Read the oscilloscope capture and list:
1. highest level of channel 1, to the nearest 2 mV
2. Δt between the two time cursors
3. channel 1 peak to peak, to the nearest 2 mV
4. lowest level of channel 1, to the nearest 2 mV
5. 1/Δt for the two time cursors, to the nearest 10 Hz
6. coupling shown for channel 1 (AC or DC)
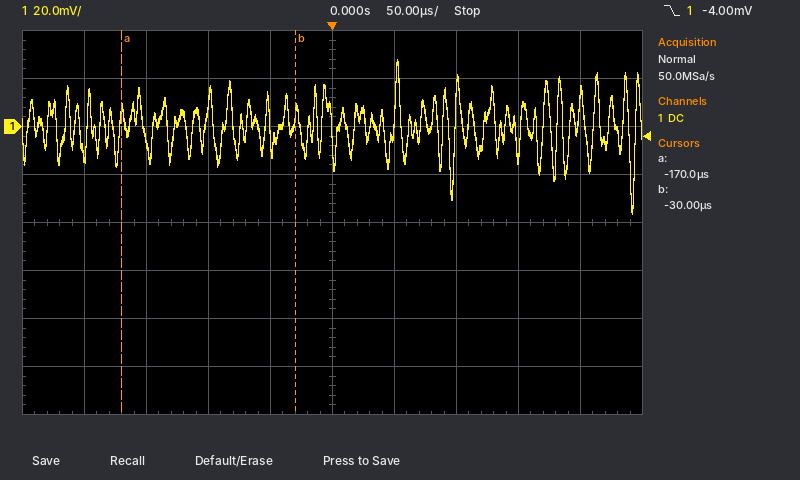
28 mV
140 µs
64 mV
-36 mV
7.14 kHz
DC
